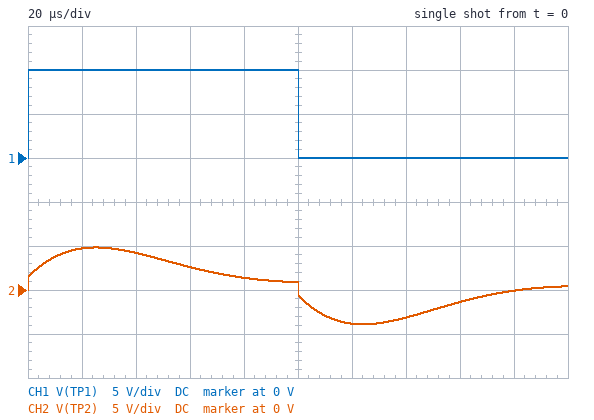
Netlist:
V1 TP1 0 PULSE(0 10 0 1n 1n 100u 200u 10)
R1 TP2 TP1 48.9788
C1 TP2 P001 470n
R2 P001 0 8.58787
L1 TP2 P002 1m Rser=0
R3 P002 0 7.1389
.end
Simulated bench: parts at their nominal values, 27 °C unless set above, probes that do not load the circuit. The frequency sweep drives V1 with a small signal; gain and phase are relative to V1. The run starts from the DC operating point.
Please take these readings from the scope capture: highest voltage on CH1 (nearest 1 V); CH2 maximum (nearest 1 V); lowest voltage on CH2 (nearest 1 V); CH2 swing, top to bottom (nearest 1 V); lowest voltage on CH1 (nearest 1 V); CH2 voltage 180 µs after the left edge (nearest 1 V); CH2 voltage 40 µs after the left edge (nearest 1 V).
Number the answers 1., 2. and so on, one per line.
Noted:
1. 10 V
2. 5 V
3. -4 V
4. 9 V
5. 0 V
6. 0 V
7. 4 V
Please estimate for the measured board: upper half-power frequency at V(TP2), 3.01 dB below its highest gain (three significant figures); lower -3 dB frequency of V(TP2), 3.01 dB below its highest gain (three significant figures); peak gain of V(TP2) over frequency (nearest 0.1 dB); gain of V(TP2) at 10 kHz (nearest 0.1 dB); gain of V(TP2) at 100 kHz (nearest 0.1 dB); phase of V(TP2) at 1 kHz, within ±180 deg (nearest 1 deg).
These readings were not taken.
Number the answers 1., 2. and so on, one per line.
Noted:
1. 12.7 kHz
2. 4.18 kHz
3. -2.6 dB
4. -3.8 dB
5. -15.9 dB
6. 34 deg
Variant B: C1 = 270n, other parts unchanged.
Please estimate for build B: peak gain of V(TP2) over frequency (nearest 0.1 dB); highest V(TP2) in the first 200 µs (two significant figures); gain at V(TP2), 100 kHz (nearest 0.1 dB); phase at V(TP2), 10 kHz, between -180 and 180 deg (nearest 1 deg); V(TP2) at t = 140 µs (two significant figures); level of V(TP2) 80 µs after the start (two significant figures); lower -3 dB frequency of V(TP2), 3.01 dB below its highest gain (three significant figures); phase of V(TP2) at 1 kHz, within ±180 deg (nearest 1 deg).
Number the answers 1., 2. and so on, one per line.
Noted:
1. -1.6 dB
2. 5.7 V
3. -14.8 dB
4. -2 deg
5. -2.4 V
6. 1.0 V
7. 5.11 kHz
8. 34 deg
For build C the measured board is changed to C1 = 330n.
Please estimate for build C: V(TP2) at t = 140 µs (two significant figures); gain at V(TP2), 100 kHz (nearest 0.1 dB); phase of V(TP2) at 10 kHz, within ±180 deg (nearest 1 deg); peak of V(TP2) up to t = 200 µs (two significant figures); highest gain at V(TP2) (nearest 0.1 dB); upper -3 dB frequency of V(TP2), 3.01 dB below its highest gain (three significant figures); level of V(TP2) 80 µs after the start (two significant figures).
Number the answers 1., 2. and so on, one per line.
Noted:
1. -2.7 V
2. -15.3 dB
3. -10 deg
4. 5.4 V
5. -1.9 dB
6. 15.8 kHz
7. 1.1 V
